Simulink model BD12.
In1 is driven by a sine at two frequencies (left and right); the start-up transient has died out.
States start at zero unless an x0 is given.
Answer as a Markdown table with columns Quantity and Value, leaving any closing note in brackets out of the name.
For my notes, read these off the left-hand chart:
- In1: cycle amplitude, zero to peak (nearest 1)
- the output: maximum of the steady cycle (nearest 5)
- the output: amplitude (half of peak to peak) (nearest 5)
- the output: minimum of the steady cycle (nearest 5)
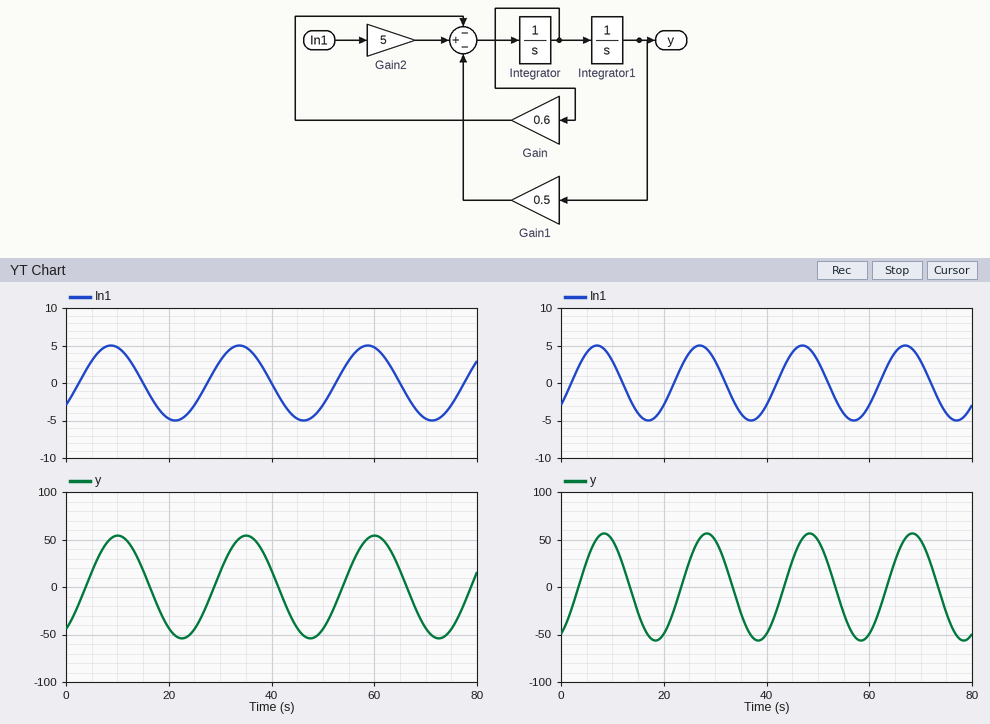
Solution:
| Quantity | Value |
|---|---|
| In1: cycle amplitude, zero to peak | 5 |
| the output: maximum of the steady cycle | 55 |
| the output: amplitude (half of peak to peak) | 55 |
| the output: minimum of the steady cycle | -55 |
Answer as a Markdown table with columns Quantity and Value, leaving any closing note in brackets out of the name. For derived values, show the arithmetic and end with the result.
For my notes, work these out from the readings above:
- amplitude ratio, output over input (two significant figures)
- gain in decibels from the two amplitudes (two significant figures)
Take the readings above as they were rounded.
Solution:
| Quantity | Value |
|---|---|
| amplitude ratio, output over input | 55 / 5 = 11 |
| gain in decibels from the two amplitudes | 20 log10(55 / 5) = 21 dB |
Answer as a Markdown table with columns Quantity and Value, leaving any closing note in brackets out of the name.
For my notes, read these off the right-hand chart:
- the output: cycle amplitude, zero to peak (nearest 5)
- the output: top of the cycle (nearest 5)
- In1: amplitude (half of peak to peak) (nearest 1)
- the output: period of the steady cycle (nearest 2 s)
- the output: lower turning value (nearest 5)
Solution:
| Quantity | Value |
|---|---|
| the output: cycle amplitude, zero to peak | 55 |
| the output: top of the cycle | 55 |
| In1: amplitude (half of peak to peak) | 5 |
| the output: period of the steady cycle | 20 s |
| the output: lower turning value | -55 |
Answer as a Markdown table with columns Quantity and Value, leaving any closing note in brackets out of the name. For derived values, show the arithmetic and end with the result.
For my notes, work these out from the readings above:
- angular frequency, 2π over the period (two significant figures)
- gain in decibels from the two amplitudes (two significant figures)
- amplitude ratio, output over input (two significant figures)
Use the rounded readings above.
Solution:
| Quantity | Value |
|---|---|
| angular frequency, 2π over the period | 2π / 20 = 0.31 rad/s |
| gain in decibels from the two amplitudes | 20 log10(55 / 5) = 21 dB |
| amplitude ratio, output over input | 55 / 5 = 11 |
